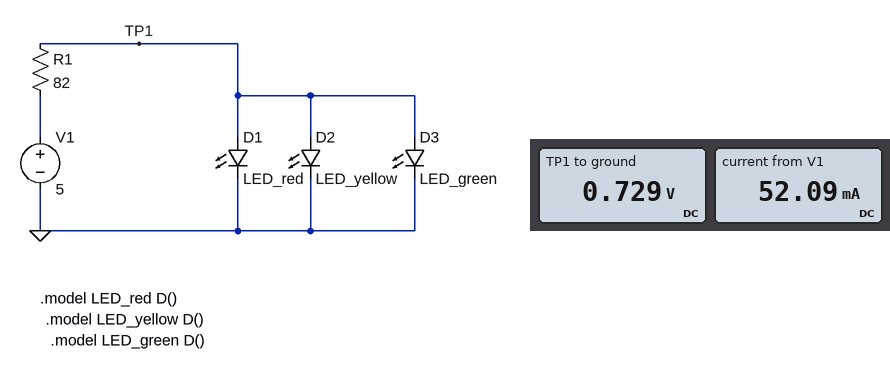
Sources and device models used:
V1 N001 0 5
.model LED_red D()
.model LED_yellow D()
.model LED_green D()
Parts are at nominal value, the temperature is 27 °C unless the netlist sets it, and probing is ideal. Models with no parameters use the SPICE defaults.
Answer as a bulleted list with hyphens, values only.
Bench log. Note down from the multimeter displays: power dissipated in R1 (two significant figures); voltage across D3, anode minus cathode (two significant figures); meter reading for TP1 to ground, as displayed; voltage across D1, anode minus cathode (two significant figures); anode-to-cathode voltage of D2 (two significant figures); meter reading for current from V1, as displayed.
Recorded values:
- 220 mW
- 730 mV
- 0.729 V
- 730 mV
- 730 mV
- 52.09 mA
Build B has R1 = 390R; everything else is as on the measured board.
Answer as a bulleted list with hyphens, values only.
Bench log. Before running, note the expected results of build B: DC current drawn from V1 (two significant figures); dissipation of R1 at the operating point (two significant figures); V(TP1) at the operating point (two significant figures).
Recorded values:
- 11 mA
- 48 mW
- 690 mV
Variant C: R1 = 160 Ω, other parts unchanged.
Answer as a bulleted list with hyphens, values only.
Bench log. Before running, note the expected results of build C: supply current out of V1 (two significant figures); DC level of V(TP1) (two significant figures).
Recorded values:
- 27 mA
- 710 mV
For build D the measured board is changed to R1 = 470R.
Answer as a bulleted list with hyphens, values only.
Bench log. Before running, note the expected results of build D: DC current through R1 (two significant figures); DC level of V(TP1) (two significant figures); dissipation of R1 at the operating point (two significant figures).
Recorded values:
- 9.2 mA
- 680 mV
- 40 mW
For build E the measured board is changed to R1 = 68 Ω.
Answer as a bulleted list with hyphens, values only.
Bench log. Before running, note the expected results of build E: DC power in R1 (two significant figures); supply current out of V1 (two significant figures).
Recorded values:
- 270 mW
- 63 mA
